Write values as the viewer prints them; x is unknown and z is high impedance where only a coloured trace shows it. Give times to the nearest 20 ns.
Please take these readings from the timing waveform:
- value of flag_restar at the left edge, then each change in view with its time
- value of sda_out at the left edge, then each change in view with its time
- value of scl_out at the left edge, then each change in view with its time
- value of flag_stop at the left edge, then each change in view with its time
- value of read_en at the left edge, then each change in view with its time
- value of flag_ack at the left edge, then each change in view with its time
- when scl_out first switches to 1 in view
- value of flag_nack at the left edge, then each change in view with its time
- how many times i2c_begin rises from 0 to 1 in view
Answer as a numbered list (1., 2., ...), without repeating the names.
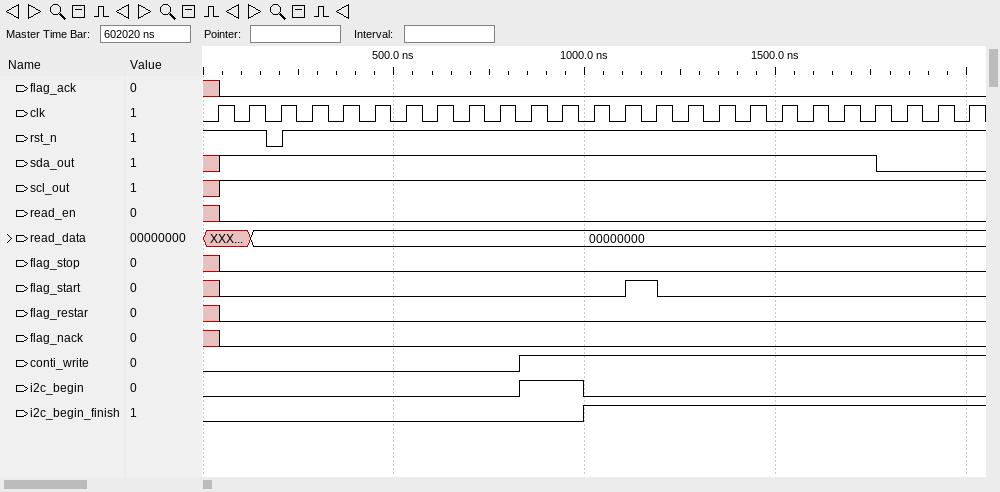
1. x, 0 at 40 ns
2. x, 1 at 40 ns, 0 at 1760 ns
3. x, 1 at 40 ns
4. x, 0 at 40 ns
5. x, 0 at 40 ns
6. x, 0 at 40 ns
7. 40 ns
8. x, 0 at 40 ns
9. 1
